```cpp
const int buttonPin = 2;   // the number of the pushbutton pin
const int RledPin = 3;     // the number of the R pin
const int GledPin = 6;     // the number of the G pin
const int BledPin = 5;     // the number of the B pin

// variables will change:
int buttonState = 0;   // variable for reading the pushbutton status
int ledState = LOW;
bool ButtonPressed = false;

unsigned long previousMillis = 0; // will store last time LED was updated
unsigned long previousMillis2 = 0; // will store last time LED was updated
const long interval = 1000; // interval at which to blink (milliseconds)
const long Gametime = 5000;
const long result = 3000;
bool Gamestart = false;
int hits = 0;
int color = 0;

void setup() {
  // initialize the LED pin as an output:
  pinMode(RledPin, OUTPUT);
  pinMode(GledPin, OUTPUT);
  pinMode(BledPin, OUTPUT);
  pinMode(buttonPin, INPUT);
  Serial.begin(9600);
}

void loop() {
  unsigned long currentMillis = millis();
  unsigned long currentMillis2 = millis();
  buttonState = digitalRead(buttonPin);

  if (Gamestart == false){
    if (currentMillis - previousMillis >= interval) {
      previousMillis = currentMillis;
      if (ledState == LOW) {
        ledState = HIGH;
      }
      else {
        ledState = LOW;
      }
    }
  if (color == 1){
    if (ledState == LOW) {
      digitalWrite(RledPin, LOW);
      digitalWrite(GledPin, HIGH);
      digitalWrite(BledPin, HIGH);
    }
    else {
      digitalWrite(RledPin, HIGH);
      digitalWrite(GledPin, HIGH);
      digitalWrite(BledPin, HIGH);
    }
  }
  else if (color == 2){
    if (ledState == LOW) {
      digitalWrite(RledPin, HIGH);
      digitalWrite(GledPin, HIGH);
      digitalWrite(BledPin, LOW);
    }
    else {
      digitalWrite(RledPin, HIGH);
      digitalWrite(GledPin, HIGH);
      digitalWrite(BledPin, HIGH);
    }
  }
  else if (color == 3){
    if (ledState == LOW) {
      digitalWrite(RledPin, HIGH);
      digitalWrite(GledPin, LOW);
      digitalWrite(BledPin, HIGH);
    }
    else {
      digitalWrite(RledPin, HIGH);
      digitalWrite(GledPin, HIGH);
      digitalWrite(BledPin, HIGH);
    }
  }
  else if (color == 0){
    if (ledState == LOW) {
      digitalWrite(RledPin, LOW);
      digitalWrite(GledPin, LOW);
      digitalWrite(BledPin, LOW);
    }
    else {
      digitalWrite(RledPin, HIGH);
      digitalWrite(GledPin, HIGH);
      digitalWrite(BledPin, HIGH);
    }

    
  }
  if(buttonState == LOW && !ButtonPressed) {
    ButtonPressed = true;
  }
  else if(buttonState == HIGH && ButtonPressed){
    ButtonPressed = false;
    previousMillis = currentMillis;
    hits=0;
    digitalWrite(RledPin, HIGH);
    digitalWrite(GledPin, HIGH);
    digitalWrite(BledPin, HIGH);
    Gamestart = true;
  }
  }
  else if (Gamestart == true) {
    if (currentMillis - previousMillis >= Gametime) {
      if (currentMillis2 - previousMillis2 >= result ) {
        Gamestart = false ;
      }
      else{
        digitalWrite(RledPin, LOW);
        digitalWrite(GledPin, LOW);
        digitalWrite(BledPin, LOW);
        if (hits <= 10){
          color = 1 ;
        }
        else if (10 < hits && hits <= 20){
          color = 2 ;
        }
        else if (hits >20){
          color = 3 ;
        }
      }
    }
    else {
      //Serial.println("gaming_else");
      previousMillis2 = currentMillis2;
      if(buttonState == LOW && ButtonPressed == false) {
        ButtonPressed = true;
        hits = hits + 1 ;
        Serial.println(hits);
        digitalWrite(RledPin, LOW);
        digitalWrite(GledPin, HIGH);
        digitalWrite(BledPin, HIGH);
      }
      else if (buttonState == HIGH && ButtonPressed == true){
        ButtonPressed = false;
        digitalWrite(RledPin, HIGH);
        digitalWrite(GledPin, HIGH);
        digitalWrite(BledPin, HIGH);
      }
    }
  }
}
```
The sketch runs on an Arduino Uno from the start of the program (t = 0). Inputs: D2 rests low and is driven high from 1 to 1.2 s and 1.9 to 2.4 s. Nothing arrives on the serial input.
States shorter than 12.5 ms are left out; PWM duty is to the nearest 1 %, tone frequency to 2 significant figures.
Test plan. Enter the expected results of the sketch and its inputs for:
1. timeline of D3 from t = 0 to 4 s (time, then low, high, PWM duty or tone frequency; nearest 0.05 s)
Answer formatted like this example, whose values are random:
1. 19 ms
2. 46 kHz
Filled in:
1. 0 s low; 1 s high; 1.2 s low; 1.9 s high; 2.4 s low
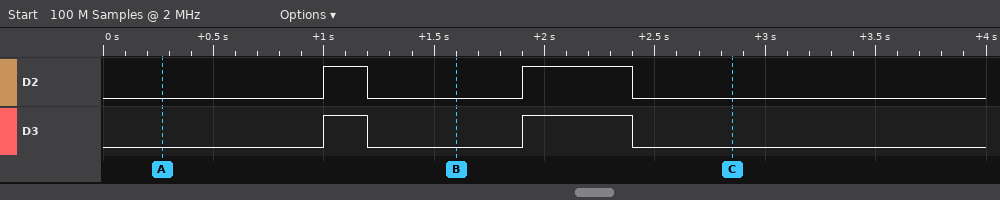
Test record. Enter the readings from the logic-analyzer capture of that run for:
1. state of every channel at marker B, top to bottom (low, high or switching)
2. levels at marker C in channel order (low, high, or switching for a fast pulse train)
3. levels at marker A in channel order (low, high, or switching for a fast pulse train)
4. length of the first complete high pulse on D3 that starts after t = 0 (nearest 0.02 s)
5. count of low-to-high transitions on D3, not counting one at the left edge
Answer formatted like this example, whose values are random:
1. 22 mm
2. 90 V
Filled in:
1. D2 low, D3 low
2. D2 low, D3 low
3. D2 low, D3 low
4. 0.20 s
5. 2
